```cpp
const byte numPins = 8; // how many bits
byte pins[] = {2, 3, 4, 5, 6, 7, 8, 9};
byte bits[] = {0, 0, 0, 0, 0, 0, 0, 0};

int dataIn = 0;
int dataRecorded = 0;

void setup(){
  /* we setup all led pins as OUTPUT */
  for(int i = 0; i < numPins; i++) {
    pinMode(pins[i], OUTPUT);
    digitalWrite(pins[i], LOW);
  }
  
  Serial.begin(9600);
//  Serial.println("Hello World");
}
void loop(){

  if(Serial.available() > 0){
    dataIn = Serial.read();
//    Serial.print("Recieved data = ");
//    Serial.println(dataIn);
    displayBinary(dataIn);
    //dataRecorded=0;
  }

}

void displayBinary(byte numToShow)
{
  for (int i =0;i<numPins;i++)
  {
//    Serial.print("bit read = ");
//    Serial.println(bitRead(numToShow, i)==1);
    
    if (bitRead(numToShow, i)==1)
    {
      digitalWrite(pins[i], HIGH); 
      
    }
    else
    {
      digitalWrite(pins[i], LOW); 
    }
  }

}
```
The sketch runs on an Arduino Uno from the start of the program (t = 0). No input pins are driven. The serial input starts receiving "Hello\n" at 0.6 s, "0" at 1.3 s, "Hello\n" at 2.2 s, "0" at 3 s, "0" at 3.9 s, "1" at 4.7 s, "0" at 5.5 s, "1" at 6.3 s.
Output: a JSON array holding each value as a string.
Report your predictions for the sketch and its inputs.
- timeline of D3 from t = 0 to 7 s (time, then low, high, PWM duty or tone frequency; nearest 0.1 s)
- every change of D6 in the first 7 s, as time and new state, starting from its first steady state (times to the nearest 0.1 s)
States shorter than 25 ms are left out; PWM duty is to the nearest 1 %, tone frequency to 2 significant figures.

["0 s low; 0.6 s high; 1.3 s low; 2.2 s high; 3 s low", "0 s low; 1.3 s high; 2.2 s low; 3 s high"]
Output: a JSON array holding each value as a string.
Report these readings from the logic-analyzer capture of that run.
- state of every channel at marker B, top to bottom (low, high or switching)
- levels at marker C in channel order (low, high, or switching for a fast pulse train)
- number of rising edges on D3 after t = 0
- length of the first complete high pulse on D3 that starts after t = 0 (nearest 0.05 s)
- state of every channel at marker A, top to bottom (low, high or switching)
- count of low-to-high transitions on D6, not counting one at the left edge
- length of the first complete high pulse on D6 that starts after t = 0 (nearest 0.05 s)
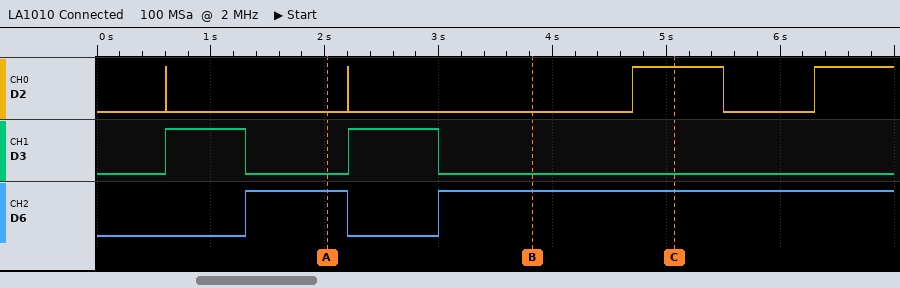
["D2 low, D3 low, D6 high", "D2 high, D3 low, D6 high", "2", "0.70 s", "D2 low, D3 low, D6 high", "2", "0.90 s"]
